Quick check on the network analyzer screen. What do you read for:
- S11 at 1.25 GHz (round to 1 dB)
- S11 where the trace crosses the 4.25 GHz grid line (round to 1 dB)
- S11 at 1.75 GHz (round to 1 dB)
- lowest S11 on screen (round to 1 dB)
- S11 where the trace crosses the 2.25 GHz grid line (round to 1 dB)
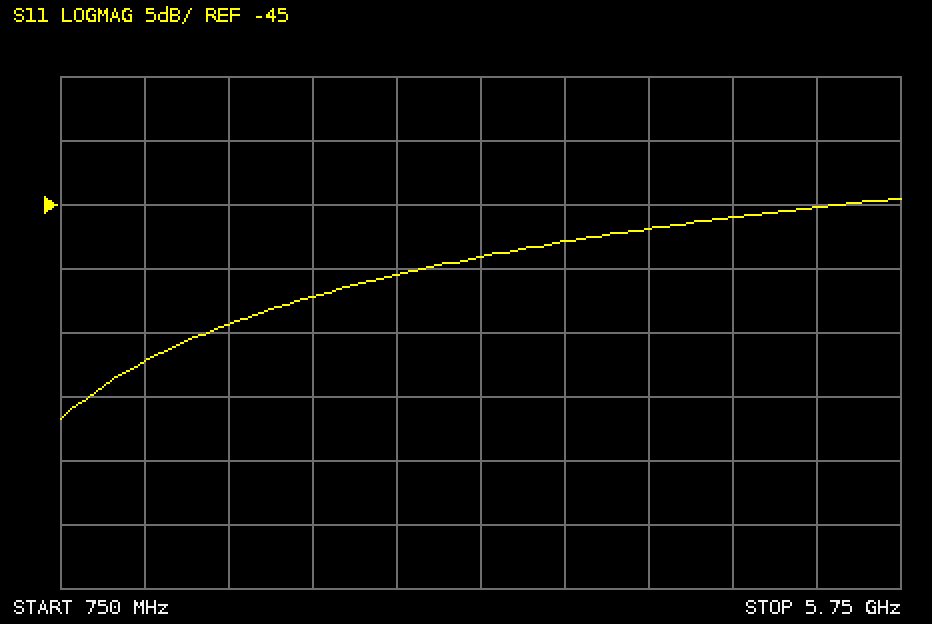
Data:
-57 dB
-47 dB
-54 dB
-62 dB
-52 dB
